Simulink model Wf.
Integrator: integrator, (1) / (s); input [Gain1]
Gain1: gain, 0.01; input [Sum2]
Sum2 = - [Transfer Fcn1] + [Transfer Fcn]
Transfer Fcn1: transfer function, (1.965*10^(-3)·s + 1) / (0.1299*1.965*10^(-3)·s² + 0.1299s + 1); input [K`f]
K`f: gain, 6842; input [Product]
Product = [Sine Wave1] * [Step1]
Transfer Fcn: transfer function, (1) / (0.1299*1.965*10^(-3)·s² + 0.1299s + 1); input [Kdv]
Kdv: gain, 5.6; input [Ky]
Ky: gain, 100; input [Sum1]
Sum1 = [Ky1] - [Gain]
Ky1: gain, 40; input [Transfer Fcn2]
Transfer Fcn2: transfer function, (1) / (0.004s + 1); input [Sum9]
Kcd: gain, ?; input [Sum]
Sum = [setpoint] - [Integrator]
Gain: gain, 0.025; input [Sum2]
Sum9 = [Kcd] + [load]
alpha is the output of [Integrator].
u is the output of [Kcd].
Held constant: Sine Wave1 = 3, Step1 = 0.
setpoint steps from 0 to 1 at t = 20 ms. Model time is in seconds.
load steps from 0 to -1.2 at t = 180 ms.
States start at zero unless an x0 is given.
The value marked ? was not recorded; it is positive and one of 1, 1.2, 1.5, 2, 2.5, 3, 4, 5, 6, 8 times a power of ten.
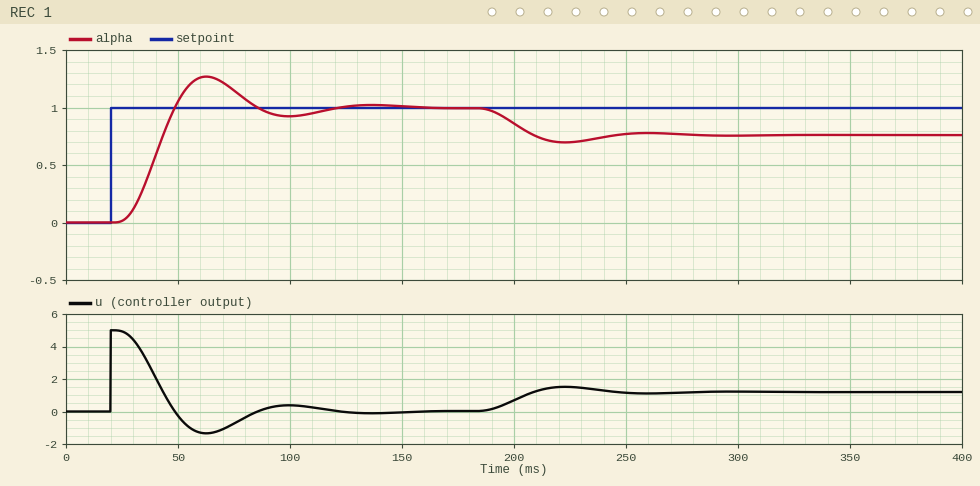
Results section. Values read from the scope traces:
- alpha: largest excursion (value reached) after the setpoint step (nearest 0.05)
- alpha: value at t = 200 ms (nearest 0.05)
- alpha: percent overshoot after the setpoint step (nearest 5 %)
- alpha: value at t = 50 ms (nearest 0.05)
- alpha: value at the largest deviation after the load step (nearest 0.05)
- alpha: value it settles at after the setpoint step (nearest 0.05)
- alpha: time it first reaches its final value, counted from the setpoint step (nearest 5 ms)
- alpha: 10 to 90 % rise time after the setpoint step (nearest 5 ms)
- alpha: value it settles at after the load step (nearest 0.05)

1.25
0.85
25 %
1.05
0.70
1.00
30 ms
15 ms
0.75
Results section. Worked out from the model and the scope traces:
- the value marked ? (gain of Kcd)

5
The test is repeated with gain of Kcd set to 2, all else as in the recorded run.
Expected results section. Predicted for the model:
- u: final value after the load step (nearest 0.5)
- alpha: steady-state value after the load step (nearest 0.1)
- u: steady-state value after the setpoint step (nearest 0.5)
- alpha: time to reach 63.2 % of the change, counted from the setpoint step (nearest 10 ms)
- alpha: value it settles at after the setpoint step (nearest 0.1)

1.0
0.4
0.0
40 ms
1.0
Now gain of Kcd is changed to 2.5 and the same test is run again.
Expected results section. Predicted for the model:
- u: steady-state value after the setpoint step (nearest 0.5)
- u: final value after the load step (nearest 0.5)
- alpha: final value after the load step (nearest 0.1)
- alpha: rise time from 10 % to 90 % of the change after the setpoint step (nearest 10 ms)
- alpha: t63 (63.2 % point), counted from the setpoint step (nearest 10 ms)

0.0
1.0
0.5
30 ms
30 ms
